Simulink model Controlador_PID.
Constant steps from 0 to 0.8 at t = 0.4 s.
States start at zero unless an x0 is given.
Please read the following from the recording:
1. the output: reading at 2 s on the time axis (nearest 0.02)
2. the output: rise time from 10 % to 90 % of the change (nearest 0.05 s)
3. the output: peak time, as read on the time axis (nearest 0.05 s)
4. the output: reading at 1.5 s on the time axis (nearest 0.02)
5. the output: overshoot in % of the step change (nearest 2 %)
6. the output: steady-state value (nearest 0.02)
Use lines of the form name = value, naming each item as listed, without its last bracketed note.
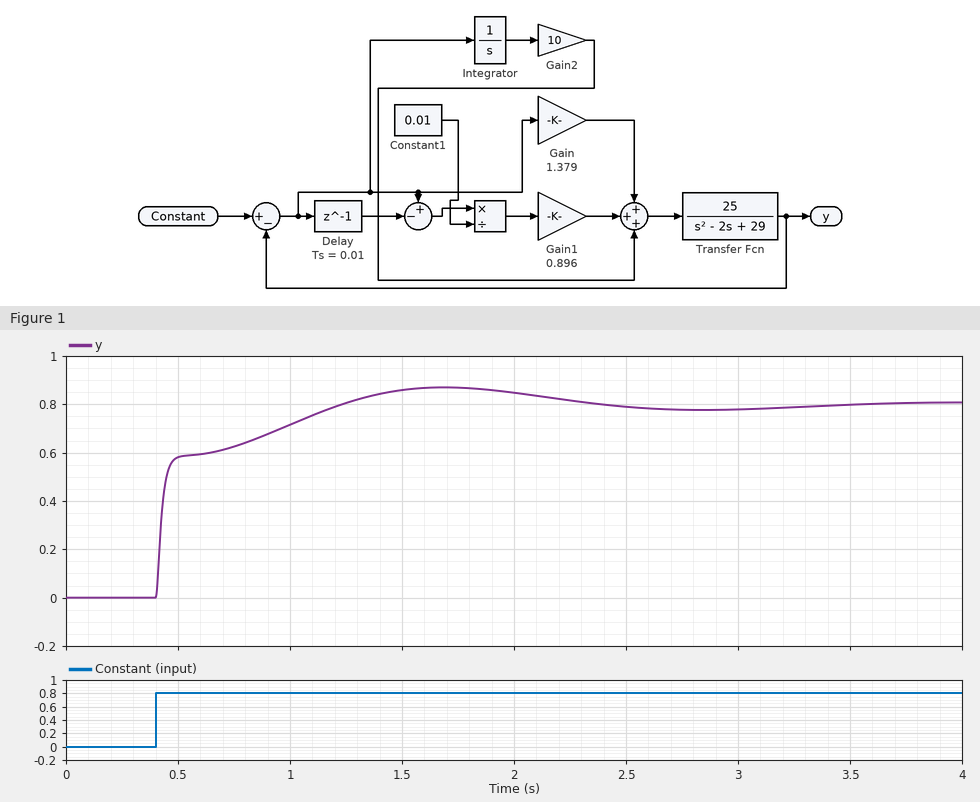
the output: reading at 2 s on the time axis = 0.84
the output: rise time from 10 % to 90 % of the change = 0.60 s
the output: peak time, as read on the time axis = 1.70 s
the output: reading at 1.5 s on the time axis = 0.86
the output: overshoot in % of the step change = 8 %
the output: steady-state value = 0.80
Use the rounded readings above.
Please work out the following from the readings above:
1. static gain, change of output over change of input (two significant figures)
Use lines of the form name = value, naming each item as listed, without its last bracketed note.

static gain, change of output over change of input = 1.0
